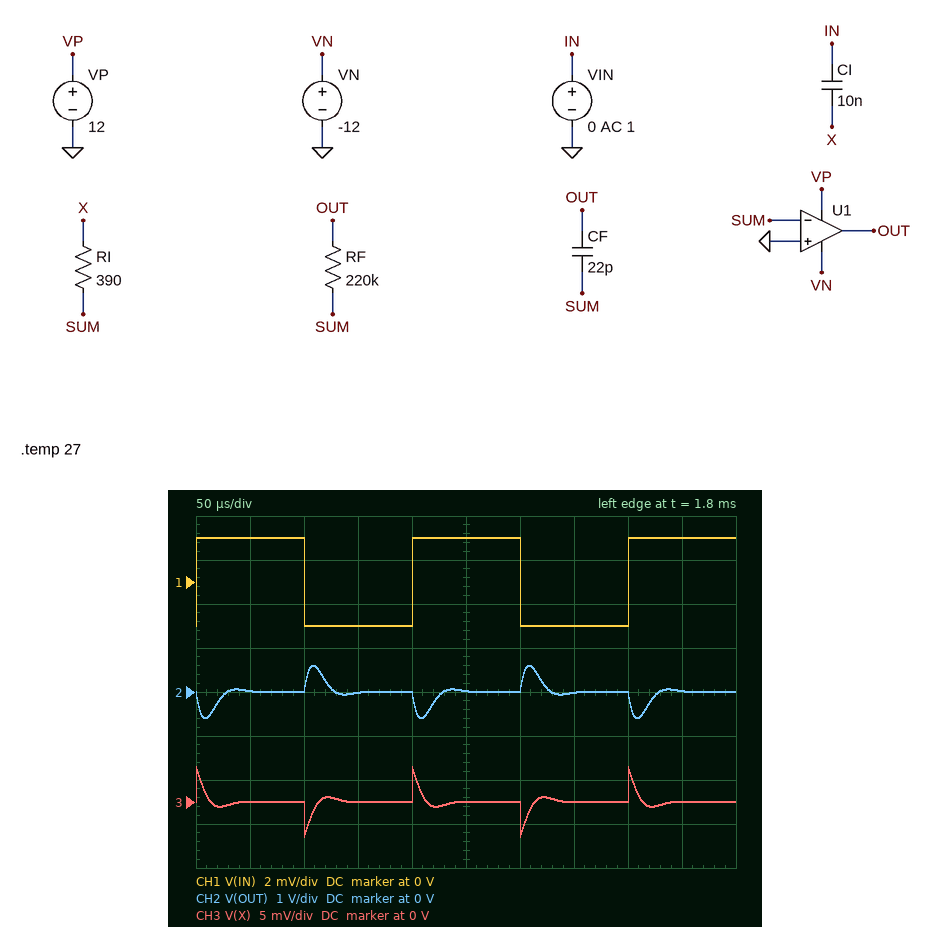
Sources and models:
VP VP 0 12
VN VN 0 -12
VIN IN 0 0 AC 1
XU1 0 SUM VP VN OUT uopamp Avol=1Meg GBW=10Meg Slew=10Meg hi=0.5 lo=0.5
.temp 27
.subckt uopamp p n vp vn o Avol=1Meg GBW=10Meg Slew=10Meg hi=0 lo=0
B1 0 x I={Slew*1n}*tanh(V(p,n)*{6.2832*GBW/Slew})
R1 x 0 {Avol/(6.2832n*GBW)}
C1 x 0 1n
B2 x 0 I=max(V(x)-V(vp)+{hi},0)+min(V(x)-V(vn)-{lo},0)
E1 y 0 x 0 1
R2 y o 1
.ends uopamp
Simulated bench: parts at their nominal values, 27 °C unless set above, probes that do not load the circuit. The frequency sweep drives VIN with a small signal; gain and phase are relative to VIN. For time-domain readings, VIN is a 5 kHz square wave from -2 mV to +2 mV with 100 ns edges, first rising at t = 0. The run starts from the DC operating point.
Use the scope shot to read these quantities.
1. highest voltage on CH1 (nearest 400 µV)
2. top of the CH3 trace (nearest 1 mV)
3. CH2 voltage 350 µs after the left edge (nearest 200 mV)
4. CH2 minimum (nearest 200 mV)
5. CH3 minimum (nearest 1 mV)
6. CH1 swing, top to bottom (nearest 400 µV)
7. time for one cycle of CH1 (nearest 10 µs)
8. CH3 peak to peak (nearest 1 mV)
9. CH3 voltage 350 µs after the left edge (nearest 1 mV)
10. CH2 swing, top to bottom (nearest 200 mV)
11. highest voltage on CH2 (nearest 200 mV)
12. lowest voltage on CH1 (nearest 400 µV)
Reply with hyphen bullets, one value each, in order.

- 2.0 mV
- 4 mV
- 0 V
- -600 mV
- -4 mV
- 4.0 mV
- 200 µs
- 8 mV
- 0 V
- 1.2 V
- 600 mV
- -2.0 mV
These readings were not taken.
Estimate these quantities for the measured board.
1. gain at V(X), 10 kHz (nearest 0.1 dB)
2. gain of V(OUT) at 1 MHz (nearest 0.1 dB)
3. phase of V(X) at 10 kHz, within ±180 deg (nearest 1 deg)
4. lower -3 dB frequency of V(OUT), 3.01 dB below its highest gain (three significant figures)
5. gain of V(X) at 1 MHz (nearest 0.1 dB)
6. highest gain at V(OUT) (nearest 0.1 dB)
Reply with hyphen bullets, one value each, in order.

- -9.4 dB
- 16.2 dB
- 96 deg
- 12.3 kHz
- 0 dB
- 48.0 dB
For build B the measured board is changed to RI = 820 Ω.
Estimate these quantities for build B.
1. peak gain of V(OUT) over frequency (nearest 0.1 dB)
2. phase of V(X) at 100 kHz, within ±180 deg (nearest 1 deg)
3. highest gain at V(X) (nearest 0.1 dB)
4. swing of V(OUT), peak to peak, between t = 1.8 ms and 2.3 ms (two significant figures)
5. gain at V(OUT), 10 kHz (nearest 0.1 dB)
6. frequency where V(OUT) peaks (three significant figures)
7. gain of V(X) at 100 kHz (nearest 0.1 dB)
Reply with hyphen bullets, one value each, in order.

- 44.5 dB
- 6 deg
- 0.3 dB
- 890 mV
- 42.1 dB
- 18.4 kHz
- 0.1 dB
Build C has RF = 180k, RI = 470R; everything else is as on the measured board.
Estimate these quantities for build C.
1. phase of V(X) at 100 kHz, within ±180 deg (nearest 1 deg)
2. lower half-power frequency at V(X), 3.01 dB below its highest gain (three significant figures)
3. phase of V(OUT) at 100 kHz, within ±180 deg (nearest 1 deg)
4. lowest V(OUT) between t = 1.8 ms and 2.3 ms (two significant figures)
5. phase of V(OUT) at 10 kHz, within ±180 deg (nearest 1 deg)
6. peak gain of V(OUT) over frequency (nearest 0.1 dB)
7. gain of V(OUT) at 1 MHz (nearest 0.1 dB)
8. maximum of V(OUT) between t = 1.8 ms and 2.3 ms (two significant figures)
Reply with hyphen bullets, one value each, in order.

- 8 deg
- 18.2 kHz
- 107 deg
- -510 mV
- -124 deg
- 46.3 dB
- 15.6 dB
- 510 mV
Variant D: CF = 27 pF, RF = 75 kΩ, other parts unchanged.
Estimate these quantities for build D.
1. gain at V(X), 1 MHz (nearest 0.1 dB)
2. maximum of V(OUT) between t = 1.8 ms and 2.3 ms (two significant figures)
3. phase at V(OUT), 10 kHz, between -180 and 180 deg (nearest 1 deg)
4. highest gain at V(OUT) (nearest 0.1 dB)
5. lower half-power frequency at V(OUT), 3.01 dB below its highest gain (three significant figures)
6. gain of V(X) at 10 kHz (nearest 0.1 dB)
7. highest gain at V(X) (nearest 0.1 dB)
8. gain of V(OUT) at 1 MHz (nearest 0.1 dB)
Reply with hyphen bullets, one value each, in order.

- 0 dB
- 320 mV
- -112 deg
- 42.0 dB
- 19.1 kHz
- -11.7 dB
- 0.9 dB
- 15.6 dB
